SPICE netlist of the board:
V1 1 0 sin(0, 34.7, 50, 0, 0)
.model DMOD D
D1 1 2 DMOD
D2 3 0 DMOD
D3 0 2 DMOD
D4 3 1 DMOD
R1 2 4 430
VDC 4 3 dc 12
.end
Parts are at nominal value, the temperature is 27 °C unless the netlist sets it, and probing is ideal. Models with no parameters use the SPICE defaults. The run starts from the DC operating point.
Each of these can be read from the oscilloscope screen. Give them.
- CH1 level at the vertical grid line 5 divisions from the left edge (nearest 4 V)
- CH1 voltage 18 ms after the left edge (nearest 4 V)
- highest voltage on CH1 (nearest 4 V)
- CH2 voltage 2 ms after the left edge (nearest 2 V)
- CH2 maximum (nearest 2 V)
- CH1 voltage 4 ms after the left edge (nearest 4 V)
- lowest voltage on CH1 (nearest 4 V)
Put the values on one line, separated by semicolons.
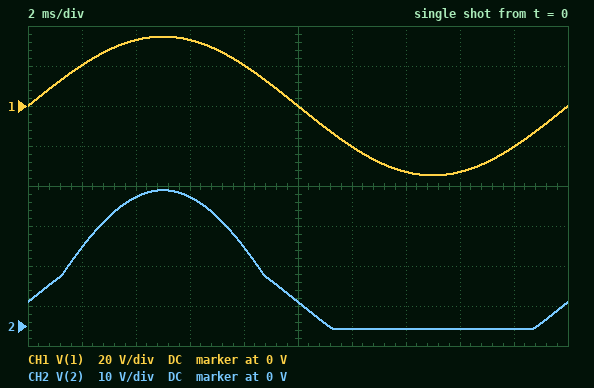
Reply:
0 V; -20 V; 36 V; 20 V; 34 V; 32 V; -36 V
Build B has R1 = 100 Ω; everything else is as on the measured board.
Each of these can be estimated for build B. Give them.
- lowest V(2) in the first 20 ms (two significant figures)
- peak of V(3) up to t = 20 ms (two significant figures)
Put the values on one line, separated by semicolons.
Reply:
-790 mV; 790 mV
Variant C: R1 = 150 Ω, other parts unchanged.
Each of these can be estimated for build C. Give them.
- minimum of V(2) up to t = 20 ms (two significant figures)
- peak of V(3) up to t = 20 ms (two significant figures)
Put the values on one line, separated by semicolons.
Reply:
-780 mV; 780 mV
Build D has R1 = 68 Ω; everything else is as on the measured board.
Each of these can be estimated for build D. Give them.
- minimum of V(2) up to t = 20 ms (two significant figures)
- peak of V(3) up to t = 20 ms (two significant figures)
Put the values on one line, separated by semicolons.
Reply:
-800 mV; 800 mV
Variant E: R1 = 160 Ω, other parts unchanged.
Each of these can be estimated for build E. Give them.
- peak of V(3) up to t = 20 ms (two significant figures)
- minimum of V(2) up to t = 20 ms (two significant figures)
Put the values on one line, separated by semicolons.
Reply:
780 mV; -780 mV
